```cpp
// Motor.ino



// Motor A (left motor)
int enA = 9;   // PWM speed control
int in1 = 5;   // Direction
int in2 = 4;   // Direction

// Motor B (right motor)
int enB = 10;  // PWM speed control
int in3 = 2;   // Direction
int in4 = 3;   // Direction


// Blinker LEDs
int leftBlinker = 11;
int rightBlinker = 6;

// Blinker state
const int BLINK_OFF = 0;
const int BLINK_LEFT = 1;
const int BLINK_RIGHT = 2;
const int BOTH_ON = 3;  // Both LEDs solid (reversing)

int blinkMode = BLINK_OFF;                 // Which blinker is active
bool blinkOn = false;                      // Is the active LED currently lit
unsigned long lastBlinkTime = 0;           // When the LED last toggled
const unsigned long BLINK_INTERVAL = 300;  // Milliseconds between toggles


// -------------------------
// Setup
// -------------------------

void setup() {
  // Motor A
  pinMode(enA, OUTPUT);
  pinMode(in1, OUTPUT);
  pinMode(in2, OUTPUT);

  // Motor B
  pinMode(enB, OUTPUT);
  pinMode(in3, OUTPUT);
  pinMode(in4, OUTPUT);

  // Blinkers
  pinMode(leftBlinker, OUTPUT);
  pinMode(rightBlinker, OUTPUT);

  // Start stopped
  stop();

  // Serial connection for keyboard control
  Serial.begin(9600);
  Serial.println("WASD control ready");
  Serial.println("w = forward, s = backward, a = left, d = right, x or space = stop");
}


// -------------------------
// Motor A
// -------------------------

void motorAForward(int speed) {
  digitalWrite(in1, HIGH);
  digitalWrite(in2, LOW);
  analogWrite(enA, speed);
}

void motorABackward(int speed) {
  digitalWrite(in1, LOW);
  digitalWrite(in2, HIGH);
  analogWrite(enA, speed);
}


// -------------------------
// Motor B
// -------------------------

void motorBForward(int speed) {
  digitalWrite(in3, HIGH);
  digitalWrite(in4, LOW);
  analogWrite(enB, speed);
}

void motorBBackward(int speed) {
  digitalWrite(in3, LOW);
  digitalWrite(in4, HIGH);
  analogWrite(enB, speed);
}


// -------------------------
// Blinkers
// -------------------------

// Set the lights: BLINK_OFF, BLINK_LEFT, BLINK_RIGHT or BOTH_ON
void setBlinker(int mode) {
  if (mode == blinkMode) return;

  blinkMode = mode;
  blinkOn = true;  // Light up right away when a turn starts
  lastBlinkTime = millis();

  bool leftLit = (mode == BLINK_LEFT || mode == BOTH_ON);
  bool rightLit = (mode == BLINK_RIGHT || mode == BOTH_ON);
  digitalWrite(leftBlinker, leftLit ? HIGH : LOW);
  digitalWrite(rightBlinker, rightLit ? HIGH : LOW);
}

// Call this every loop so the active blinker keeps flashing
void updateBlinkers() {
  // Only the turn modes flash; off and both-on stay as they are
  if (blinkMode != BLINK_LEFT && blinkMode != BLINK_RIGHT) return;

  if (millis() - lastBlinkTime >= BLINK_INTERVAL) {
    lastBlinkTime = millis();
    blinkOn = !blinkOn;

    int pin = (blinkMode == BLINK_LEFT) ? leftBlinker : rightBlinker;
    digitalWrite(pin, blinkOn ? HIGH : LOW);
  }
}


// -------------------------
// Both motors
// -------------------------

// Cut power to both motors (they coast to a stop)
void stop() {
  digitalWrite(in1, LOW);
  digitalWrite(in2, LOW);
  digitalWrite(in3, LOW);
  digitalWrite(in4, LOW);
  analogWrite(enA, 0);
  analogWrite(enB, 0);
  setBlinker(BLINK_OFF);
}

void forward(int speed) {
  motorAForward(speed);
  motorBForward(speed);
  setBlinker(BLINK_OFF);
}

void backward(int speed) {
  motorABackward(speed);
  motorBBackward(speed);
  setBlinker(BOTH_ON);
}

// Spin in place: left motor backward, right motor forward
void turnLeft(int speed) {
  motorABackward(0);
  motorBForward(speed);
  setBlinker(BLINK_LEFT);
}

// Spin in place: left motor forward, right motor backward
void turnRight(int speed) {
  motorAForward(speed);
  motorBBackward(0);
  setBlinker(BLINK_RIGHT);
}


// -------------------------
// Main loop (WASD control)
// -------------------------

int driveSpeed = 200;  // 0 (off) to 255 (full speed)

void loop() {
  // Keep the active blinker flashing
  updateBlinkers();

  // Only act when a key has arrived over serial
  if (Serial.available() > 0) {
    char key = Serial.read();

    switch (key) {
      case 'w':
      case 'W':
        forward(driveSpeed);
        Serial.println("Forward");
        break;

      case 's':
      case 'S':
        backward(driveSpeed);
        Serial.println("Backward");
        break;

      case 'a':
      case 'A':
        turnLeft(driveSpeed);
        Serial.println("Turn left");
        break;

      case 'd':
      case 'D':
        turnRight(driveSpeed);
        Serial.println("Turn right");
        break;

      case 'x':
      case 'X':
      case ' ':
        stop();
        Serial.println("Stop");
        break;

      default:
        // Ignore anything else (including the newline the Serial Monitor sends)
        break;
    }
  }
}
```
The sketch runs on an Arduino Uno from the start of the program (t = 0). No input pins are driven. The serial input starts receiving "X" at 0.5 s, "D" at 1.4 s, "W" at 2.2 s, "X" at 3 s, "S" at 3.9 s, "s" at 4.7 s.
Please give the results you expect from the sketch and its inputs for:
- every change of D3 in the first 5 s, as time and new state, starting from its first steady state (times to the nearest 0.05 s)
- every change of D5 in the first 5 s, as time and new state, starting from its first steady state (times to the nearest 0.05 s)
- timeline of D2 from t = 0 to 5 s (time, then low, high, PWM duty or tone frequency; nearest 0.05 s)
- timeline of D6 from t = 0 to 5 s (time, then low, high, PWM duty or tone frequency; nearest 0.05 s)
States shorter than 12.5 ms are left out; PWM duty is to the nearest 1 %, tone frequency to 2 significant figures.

0 s low; 1.4 s high; 2.2 s low; 3.9 s high
0 s low; 1.4 s high; 3 s low
0 s low; 2.2 s high; 3 s low
0 s low; 1.4 s high; 1.7 s low; 2 s high; 2.2 s low; 3.9 s high
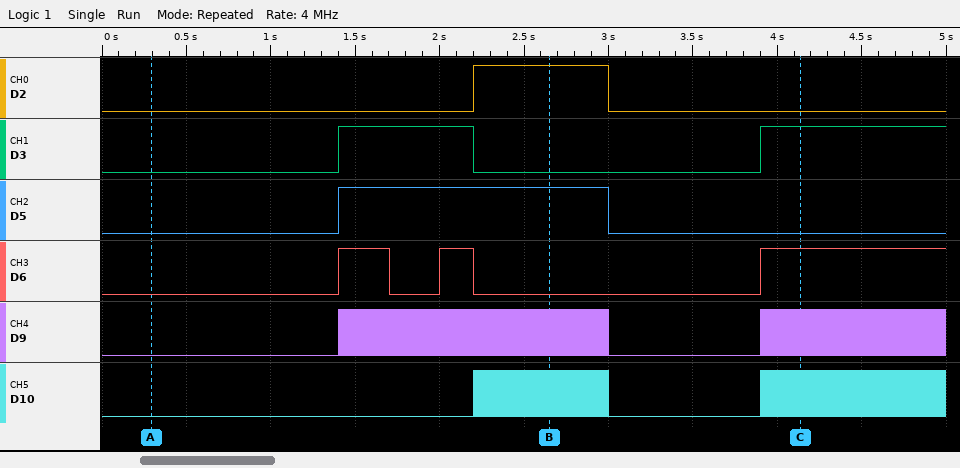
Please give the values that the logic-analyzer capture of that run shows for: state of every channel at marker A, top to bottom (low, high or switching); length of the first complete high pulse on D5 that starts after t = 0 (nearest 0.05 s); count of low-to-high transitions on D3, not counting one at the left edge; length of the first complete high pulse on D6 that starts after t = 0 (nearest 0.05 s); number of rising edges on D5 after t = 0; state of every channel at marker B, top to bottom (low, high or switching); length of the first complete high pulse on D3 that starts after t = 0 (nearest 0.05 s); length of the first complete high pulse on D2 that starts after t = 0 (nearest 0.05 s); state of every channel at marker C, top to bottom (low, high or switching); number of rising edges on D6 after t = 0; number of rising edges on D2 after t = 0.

D2 low, D3 low, D5 low, D6 low, D9 low, D10 low
1.60 s
2
0.30 s
1
D2 high, D3 low, D5 high, D6 low, D9 switching, D10 switching
0.80 s
0.80 s
D2 low, D3 high, D5 low, D6 high, D9 switching, D10 switching
3
1
